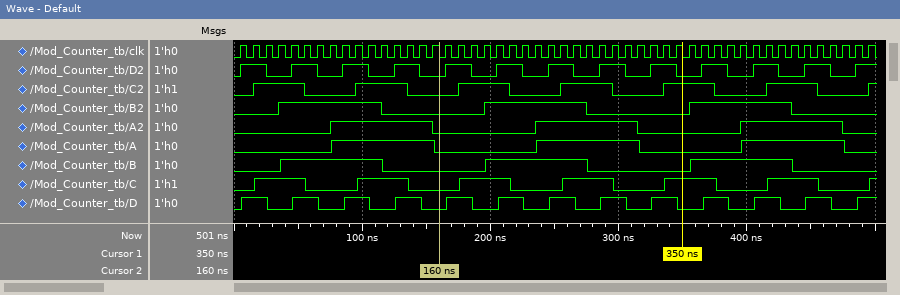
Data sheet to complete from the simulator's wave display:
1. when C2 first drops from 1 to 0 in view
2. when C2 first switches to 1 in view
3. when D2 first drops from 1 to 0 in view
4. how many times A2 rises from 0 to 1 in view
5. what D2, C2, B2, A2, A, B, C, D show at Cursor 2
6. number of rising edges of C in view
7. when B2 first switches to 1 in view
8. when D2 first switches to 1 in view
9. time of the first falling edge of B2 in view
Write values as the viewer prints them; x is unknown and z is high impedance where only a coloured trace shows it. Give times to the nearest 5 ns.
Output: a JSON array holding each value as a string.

["55 ns", "15 ns", "25 ns", "3", "D2=0, C2=0, B2=0, A2=0, A=0, B=0, C=0, D=0", "7", "35 ns", "5 ns", "115 ns"]
